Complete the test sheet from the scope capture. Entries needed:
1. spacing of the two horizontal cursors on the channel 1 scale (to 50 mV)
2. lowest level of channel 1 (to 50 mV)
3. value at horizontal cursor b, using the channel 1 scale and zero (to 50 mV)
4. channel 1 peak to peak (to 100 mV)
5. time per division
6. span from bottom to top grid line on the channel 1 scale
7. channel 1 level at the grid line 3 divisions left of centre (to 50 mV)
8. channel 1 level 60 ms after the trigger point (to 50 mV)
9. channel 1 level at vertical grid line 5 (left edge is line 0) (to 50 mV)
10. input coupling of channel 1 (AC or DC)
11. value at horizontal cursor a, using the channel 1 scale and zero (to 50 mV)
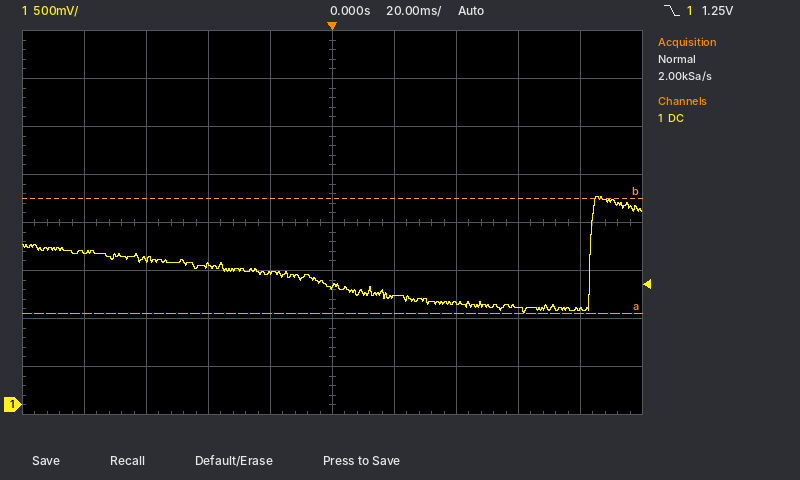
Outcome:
1.20 V
950 mV
2.15 V
1.20 V
20 ms
4 V
1.50 V
1.00 V
1.25 V
DC
950 mV
